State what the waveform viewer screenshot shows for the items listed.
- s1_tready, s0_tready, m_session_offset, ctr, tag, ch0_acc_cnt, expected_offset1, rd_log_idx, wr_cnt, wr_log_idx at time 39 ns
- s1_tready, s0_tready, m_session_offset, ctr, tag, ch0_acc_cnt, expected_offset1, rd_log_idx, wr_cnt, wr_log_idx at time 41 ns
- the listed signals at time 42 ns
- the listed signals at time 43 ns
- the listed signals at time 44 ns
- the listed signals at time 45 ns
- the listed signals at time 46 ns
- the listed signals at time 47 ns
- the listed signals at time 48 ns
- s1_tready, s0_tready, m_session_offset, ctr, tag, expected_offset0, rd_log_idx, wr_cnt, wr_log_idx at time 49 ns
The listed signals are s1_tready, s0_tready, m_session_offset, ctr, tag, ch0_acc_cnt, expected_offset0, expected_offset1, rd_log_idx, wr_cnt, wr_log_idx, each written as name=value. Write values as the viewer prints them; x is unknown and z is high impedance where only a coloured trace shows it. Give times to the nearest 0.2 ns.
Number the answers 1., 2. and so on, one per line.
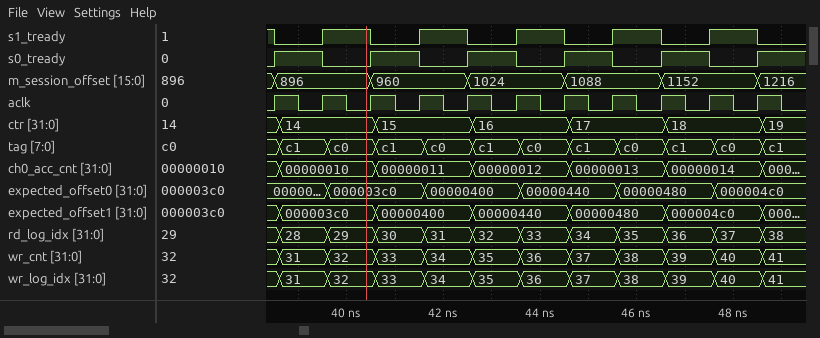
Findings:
1. s1_tready=0, s0_tready=1, m_session_offset=896, ctr=14, tag=c1, ch0_acc_cnt=00000010, expected_offset1=000003c0, rd_log_idx=28, wr_cnt=31, wr_log_idx=31
2. s1_tready=0, s0_tready=1, m_session_offset=960, ctr=15, tag=c1, ch0_acc_cnt=00000011, expected_offset1=00000400, rd_log_idx=30, wr_cnt=33, wr_log_idx=33
3. s1_tready=1, s0_tready=0, m_session_offset=960, ctr=15, tag=c0, ch0_acc_cnt=00000011, expected_offset0=00000400, expected_offset1=00000400, rd_log_idx=31, wr_cnt=34, wr_log_idx=34
4. s1_tready=0, s0_tready=1, m_session_offset=1024, ctr=16, tag=c1, ch0_acc_cnt=00000012, expected_offset0=00000400, expected_offset1=00000440, rd_log_idx=32, wr_cnt=35, wr_log_idx=35
5. s1_tready=1, s0_tready=0, m_session_offset=1024, ctr=16, tag=c0, ch0_acc_cnt=00000012, expected_offset0=00000440, expected_offset1=00000440, rd_log_idx=33, wr_cnt=36, wr_log_idx=36
6. s1_tready=0, s0_tready=1, m_session_offset=1088, ctr=17, tag=c1, ch0_acc_cnt=00000013, expected_offset0=00000440, expected_offset1=00000480, rd_log_idx=34, wr_cnt=37, wr_log_idx=37
7. s1_tready=1, s0_tready=0, m_session_offset=1088, ctr=17, tag=c0, ch0_acc_cnt=00000013, expected_offset0=00000480, expected_offset1=00000480, rd_log_idx=35, wr_cnt=38, wr_log_idx=38
8. s1_tready=0, s0_tready=1, m_session_offset=1152, ctr=18, tag=c1, ch0_acc_cnt=00000014, expected_offset0=00000480, expected_offset1=000004c0, rd_log_idx=36, wr_cnt=39, wr_log_idx=39
9. s1_tready=1, s0_tready=0, m_session_offset=1152, ctr=18, tag=c0, ch0_acc_cnt=00000014, expected_offset0=000004c0, expected_offset1=000004c0, rd_log_idx=37, wr_cnt=40, wr_log_idx=40
10. s1_tready=0, s0_tready=1, m_session_offset=1216, ctr=19, tag=c1, expected_offset0=000004c0, rd_log_idx=38, wr_cnt=41, wr_log_idx=41
